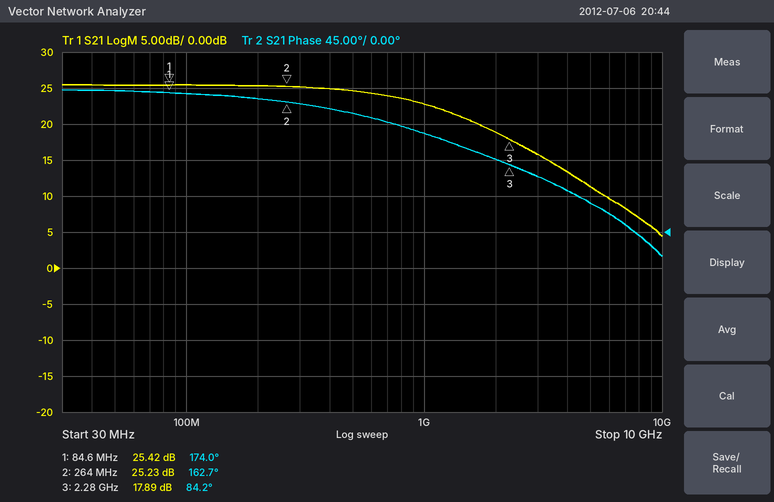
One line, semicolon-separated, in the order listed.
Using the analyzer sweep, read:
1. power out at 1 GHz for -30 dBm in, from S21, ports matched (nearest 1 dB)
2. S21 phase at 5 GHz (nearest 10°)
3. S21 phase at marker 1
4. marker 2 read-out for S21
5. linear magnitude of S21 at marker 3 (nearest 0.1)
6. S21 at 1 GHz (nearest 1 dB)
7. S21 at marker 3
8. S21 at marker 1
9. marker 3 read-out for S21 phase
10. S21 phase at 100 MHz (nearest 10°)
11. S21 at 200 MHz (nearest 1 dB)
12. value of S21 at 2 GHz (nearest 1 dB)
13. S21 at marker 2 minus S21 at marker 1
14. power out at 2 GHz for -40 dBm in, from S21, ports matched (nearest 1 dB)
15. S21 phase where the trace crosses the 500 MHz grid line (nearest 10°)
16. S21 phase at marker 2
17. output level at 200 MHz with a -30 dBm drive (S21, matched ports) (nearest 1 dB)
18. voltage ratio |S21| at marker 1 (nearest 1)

-7 dBm; 40°; 174.0°; 25.23 dB; 7.8; 23 dB; 17.89 dB; 25.42 dB; 84.2°; 170°; 25 dB; 19 dB; -0.19 dB; -21 dBm; 150°; 162.7°; -5 dBm; 19
